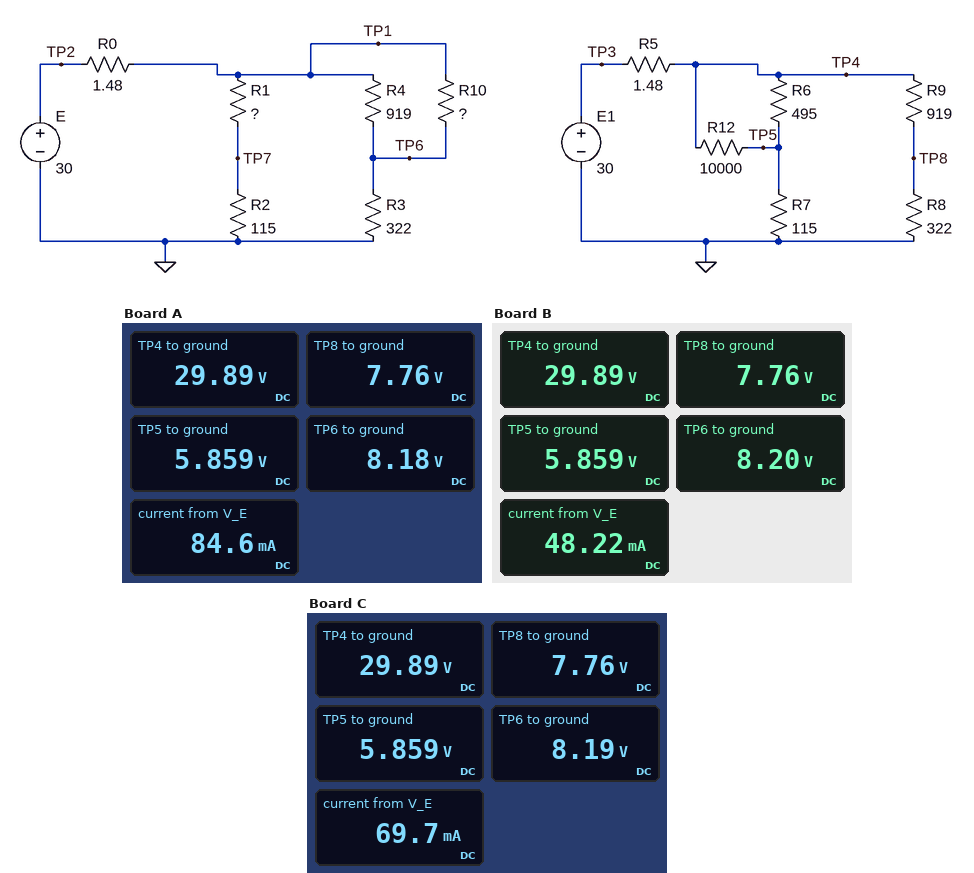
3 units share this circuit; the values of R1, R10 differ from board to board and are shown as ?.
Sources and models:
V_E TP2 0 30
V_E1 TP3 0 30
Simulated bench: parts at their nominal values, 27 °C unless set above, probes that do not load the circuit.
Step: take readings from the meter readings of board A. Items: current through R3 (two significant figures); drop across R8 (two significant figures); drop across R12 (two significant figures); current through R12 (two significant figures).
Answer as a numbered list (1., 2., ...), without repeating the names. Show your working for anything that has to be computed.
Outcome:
1. (8.18 V) / 322 Ω = 25 mA
2. 7.76 V = 7.8 V
3. 29.89 V - 5.859 V = 24 V
4. (29.89 V - 5.859 V) / 10 kΩ = 2.4 mA
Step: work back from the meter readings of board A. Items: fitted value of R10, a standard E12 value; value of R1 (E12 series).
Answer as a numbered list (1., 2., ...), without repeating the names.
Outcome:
1. 12 kΩ
2. 390 Ω
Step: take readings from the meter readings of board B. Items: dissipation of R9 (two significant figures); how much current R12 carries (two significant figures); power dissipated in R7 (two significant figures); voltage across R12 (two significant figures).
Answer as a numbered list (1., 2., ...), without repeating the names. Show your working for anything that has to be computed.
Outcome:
1. (29.89 V - 7.76 V)^2 / 919 Ω = 530 mW
2. (29.89 V - 5.859 V) / 10 kΩ = 2.4 mA
3. (5.859 V)^2 / 115 Ω = 300 mW
4. 29.89 V - 5.859 V = 24 V
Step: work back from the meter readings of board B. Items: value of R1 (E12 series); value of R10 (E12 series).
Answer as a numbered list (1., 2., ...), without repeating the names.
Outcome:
1. 1.2 kΩ
2. 12 kΩ
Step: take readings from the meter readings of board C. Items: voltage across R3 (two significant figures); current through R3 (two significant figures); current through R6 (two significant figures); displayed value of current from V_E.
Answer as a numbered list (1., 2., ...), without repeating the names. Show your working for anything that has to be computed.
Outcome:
1. 8.19 V = 8.2 V
2. (8.19 V) / 322 Ω = 25 mA
3. (29.89 V - 5.859 V) / 495 Ω = 49 mA
4. 69.7 mA
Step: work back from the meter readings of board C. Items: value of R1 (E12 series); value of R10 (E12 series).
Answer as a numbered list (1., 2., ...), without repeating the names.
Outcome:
1. 560 Ω
2. 12 kΩ
